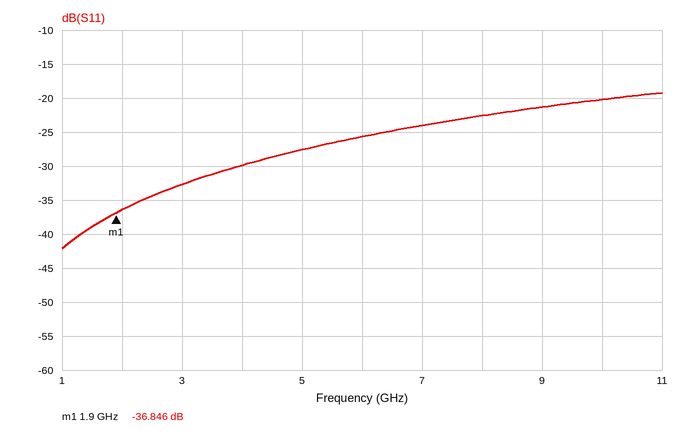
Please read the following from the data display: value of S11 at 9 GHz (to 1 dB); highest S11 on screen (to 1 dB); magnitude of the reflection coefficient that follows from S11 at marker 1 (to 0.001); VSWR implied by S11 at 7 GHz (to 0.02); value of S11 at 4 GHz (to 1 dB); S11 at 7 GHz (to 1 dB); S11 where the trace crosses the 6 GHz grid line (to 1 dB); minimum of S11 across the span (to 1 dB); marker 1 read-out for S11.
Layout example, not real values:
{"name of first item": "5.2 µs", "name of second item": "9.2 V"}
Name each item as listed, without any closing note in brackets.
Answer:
{"value of S11 at 9 GHz": "-21 dB", "highest S11 on screen": "-19 dB", "magnitude of the reflection coefficient that follows from S11 at marker 1": "0.014", "VSWR implied by S11 at 7 GHz": "1.14", "value of S11 at 4 GHz": "-30 dB", "S11 at 7 GHz": "-24 dB", "S11 where the trace crosses the 6 GHz grid line": "-26 dB", "minimum of S11 across the span": "-42 dB", "marker 1 read-out for S11": "-36.846 dB"}
